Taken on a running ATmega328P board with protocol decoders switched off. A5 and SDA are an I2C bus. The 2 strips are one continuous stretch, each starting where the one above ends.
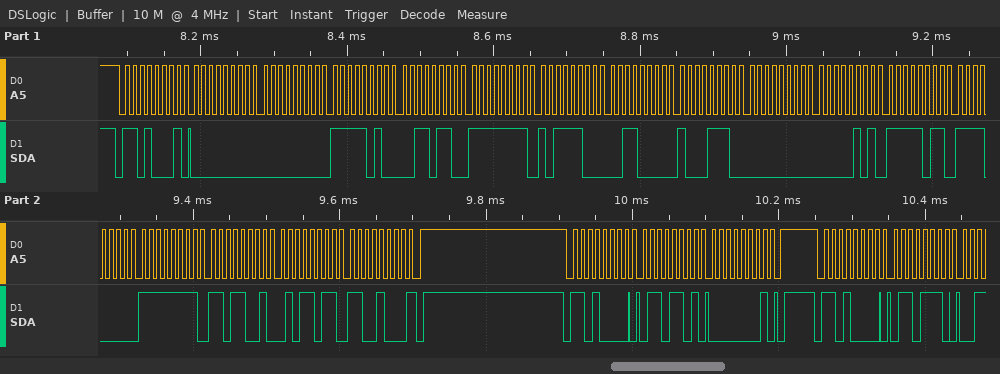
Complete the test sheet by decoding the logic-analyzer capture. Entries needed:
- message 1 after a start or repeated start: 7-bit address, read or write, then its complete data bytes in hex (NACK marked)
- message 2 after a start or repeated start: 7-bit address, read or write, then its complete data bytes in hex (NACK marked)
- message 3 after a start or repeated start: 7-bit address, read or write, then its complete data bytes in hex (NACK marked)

0x68 read: 00 00 FA 36 FF BC 30 8E 00 05 FB F0 FF D9 5B C8 NACK
0x68 write: 6D 01
0x68 write: 6E
